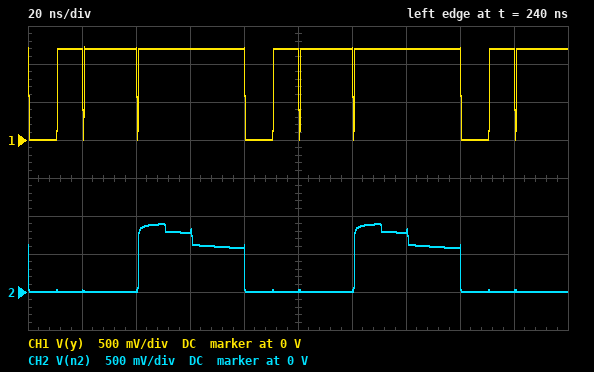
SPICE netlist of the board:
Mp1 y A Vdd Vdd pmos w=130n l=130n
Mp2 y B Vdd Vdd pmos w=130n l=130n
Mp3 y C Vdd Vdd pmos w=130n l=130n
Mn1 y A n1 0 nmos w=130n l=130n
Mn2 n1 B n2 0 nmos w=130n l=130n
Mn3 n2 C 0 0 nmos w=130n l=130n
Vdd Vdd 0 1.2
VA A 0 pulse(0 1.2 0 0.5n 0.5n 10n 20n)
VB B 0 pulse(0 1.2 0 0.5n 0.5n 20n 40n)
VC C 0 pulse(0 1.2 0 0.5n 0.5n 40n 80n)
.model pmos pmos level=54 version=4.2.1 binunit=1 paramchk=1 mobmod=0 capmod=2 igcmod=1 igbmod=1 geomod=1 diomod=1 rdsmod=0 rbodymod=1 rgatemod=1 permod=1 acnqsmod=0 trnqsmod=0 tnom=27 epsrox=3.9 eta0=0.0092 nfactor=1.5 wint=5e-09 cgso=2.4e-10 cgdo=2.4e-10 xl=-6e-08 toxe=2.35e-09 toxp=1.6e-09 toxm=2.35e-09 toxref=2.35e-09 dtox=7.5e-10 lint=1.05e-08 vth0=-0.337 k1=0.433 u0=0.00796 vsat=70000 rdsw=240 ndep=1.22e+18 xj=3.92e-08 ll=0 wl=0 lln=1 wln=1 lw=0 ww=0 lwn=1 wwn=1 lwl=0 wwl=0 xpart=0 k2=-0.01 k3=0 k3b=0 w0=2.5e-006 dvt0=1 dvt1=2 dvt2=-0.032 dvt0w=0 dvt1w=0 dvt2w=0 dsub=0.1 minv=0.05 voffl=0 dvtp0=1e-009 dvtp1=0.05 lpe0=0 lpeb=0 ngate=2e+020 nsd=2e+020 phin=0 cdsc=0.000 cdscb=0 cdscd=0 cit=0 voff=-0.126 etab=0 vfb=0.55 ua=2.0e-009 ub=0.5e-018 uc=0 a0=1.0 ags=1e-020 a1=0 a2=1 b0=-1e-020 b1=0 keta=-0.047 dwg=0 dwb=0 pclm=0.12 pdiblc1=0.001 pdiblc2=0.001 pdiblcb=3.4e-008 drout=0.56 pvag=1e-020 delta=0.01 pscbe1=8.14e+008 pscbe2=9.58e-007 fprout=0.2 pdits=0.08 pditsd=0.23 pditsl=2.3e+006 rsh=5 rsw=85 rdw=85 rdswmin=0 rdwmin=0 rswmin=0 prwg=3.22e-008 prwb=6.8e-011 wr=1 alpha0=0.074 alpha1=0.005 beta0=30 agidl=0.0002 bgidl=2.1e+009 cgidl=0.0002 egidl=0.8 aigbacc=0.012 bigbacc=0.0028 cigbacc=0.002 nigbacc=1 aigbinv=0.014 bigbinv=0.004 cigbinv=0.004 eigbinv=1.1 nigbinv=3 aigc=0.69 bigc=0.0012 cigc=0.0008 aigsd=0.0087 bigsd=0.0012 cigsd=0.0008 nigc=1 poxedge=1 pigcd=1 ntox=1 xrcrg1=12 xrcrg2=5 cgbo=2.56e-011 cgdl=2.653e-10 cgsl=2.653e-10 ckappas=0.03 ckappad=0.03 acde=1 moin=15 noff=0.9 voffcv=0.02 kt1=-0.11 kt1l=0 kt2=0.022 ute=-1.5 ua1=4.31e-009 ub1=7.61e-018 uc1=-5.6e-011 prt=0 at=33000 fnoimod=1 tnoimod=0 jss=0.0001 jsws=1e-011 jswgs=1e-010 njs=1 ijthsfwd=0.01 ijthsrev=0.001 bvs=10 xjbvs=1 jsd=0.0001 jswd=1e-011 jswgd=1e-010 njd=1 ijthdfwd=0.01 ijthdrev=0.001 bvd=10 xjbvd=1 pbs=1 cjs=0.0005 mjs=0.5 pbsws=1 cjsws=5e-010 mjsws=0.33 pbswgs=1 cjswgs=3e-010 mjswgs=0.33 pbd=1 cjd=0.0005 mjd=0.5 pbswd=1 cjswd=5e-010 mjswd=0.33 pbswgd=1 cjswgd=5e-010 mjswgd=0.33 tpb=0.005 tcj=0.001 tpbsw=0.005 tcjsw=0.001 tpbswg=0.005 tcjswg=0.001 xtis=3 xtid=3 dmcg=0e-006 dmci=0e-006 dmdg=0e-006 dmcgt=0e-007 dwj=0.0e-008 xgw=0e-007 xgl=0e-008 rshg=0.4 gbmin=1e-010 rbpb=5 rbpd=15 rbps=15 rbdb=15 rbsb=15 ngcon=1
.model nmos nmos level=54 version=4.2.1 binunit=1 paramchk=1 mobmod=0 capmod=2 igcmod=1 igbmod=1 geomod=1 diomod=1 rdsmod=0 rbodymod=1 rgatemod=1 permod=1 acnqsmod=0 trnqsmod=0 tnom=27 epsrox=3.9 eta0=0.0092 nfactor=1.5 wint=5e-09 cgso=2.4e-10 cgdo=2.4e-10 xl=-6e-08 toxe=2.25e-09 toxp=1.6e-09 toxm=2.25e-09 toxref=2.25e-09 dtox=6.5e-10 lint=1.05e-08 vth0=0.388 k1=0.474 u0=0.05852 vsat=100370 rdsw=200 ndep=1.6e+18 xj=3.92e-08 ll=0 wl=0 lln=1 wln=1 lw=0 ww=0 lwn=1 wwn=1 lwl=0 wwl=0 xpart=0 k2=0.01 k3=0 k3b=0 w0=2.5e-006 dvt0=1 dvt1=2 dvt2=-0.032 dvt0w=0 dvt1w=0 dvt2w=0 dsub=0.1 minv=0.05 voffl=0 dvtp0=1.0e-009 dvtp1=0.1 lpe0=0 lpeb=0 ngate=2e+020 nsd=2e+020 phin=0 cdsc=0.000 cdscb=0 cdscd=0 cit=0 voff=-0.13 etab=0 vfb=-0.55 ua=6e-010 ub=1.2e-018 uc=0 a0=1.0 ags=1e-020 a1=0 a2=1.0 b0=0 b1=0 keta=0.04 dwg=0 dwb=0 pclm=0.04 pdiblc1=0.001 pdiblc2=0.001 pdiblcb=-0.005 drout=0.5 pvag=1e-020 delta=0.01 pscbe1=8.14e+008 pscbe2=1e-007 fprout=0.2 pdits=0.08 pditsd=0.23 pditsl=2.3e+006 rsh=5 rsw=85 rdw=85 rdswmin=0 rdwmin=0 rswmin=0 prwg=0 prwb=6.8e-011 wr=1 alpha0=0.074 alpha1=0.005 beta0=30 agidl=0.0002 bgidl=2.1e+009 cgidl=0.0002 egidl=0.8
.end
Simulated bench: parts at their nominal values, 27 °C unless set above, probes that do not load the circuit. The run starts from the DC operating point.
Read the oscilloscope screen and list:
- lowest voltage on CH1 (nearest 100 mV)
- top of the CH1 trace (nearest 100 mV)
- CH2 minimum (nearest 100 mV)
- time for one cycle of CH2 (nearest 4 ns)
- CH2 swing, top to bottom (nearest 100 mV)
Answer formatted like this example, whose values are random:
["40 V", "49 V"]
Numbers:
["0 V", "1.2 V", "0 V", "80 ns", "900 mV"]
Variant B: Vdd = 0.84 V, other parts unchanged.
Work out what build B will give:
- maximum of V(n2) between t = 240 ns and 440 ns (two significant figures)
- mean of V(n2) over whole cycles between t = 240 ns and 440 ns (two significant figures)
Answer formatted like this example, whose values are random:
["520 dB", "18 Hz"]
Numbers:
["840 mV", "330 mV"]
